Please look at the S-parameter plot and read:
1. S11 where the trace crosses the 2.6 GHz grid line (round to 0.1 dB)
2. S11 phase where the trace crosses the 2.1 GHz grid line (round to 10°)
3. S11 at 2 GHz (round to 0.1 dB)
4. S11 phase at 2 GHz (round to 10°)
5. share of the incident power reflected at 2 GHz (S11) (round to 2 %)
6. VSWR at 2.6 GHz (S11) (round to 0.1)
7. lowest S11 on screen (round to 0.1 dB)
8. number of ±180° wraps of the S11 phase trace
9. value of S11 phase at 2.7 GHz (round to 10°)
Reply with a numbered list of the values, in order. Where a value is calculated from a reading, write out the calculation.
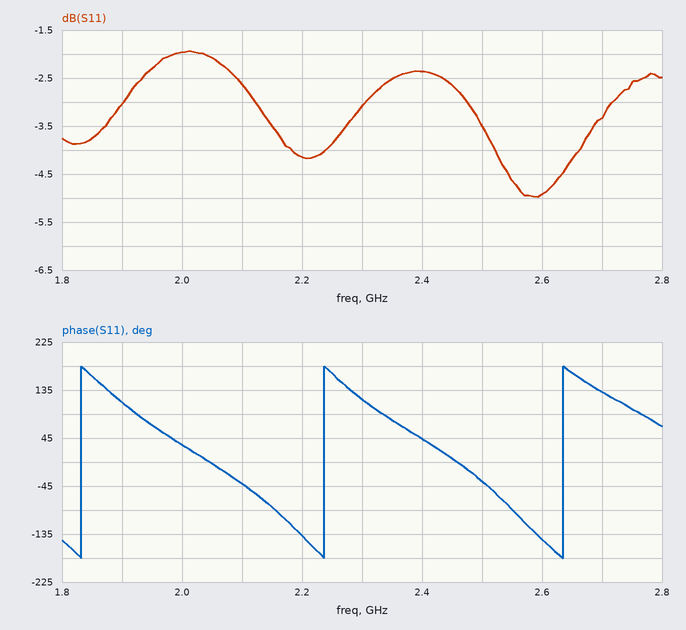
1. -4.9 dB
2. -40°
3. -2.0 dB
4. 30°
5. 10^(-2/10) ≈ 63.1 %, so 64 % to the nearest 2 %
6. |Γ| = 10^(-4.9/20) = 0.5689; VSWR = (1 + 0.5689)/(1 − 0.5689) ≈ 3.6
7. -5.0 dB
8. 3
9. 130°
